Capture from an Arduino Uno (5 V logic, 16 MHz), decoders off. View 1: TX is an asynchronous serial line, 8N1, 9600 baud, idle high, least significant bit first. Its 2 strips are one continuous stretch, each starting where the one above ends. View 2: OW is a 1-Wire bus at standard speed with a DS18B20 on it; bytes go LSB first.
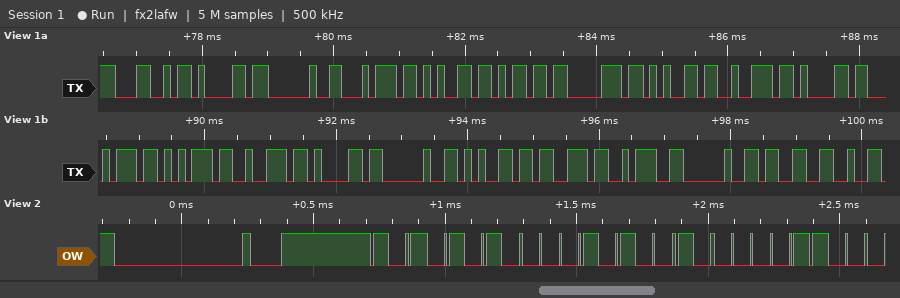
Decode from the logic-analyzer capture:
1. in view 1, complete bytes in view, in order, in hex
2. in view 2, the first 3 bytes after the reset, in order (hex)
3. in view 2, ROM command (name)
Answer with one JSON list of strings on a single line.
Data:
["0x4C 0x61 0x20 0x74 0x65 0x6D 0x70 0x65 0x72 0x61 0x74 0x75 0x72 0x61 0x20 0x65 0x73 0x3A 0x20 0x33", "55 28 C1", "Match ROM"]
